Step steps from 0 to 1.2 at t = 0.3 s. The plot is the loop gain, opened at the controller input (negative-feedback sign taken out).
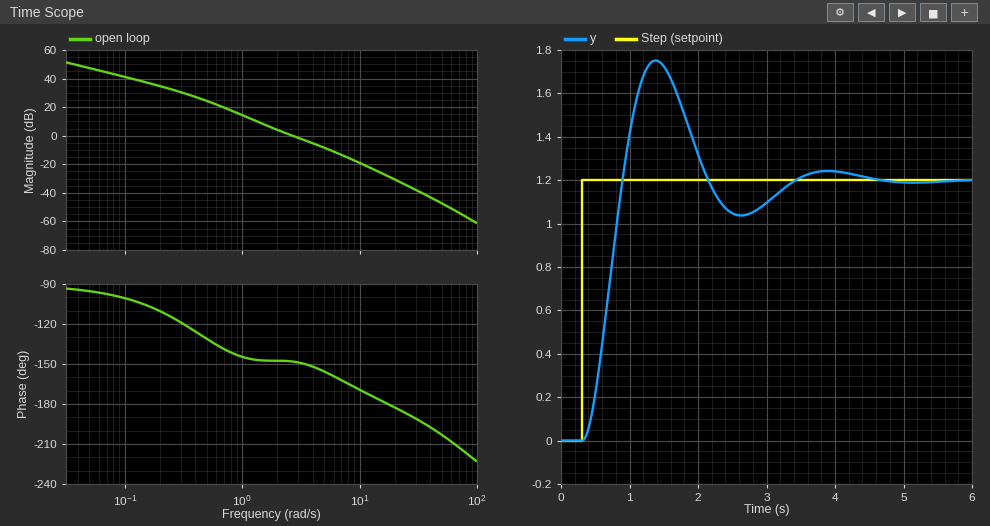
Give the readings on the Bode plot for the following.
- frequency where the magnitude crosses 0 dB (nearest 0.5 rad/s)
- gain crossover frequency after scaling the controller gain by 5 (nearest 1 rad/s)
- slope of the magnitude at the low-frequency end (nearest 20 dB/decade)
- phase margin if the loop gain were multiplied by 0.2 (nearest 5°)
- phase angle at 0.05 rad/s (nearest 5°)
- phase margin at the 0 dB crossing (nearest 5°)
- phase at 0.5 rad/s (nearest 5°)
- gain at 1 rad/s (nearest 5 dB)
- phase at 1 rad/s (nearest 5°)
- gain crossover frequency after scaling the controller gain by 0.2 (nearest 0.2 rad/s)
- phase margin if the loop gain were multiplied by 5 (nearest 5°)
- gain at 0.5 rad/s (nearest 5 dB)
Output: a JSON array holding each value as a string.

["2.5 rad/s", "7 rad/s", "-20 dB/decade", "35°", "-95°", "30°", "-130°", "15 dB", "-145°", "1.0 rad/s", "15°", "25 dB"]
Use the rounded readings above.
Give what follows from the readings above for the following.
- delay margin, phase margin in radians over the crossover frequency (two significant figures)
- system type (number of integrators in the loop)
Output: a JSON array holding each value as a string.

["0.21 s", "1"]
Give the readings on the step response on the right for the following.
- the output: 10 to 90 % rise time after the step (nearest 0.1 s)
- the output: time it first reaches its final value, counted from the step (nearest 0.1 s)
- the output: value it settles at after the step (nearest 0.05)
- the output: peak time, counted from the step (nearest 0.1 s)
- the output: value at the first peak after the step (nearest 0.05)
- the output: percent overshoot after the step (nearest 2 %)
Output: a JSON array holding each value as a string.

["0.4 s", "0.6 s", "1.20", "1.1 s", "1.75", "46 %"]
